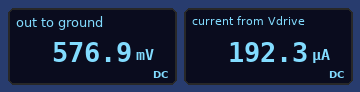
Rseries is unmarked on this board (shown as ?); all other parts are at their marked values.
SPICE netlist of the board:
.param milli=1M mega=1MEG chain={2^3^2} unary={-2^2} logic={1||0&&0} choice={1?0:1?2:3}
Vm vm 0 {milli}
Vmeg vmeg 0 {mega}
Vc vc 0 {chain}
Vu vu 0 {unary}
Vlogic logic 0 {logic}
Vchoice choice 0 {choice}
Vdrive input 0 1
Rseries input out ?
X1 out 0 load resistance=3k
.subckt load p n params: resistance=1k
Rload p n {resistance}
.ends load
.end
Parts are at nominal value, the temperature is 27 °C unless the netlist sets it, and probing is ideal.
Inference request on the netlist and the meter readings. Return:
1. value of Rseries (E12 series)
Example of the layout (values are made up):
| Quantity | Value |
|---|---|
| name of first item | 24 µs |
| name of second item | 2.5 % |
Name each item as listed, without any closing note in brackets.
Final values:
| Quantity | Value |
|---|---|
| value of Rseries | 2.2 kΩ |
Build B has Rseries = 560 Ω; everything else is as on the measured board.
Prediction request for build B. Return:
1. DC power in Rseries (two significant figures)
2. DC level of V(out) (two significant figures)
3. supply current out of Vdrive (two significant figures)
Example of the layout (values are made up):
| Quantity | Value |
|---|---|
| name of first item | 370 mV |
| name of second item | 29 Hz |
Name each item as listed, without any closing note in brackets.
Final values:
| Quantity | Value |
|---|---|
| DC power in Rseries | 44 µW |
| DC level of V(out) | 840 mV |
| supply current out of Vdrive | 280 µA |
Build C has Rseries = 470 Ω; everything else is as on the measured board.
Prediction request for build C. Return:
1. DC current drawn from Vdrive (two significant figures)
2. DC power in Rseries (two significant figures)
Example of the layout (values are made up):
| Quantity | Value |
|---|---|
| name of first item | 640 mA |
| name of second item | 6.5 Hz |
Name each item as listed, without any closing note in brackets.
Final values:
| Quantity | Value |
|---|---|
| DC current drawn from Vdrive | 290 µA |
| DC power in Rseries | 39 µW |
